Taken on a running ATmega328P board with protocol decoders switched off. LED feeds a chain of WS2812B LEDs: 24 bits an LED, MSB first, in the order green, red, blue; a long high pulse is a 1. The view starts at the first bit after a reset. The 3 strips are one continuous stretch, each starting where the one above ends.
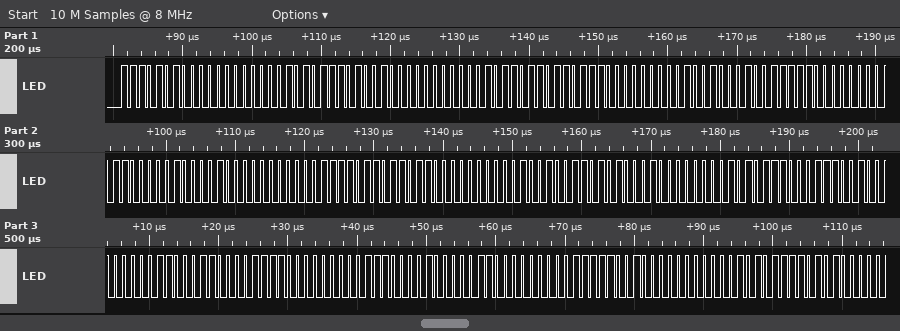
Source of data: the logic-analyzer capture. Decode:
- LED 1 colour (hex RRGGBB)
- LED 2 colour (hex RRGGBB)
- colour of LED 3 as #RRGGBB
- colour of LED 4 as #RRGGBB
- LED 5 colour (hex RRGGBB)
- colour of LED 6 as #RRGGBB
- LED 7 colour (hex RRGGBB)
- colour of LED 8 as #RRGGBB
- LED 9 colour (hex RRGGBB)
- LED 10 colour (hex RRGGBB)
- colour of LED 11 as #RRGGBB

#00EA15
#00D22D
#00B748
#009F60
#00847B
#006C93
#0051AE
#0039C6
#001EE1
#0006F9
#1500EA
